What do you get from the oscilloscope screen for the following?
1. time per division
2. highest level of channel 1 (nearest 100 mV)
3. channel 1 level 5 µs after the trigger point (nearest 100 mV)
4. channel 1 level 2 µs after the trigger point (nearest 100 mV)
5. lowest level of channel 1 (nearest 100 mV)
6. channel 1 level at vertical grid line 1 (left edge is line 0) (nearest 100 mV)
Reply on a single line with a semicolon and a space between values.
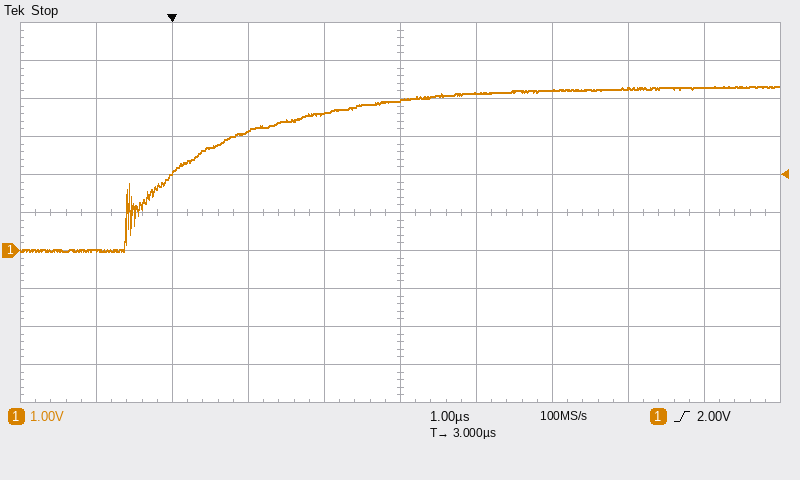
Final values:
1 µs; 4.3 V; 4.2 V; 3.6 V; 0.0 V; 0.0 V
